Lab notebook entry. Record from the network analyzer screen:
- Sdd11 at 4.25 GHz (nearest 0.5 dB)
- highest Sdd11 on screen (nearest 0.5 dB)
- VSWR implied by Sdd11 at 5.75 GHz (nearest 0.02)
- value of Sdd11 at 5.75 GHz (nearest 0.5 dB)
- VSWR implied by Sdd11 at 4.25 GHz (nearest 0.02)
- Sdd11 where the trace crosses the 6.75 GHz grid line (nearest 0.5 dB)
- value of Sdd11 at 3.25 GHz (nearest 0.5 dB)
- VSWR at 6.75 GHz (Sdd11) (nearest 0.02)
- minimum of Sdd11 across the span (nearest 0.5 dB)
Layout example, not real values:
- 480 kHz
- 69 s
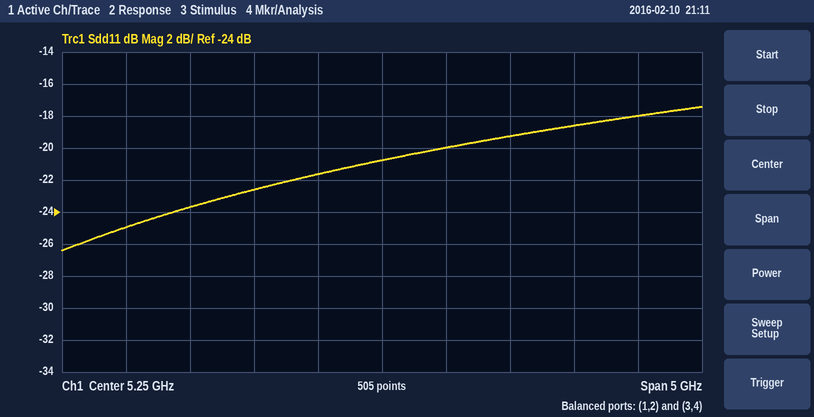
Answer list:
- -22.5 dB
- -17.5 dB
- 1.22
- -20.0 dB
- 1.16
- -18.5 dB
- -25.0 dB
- 1.26
- -26.5 dB
